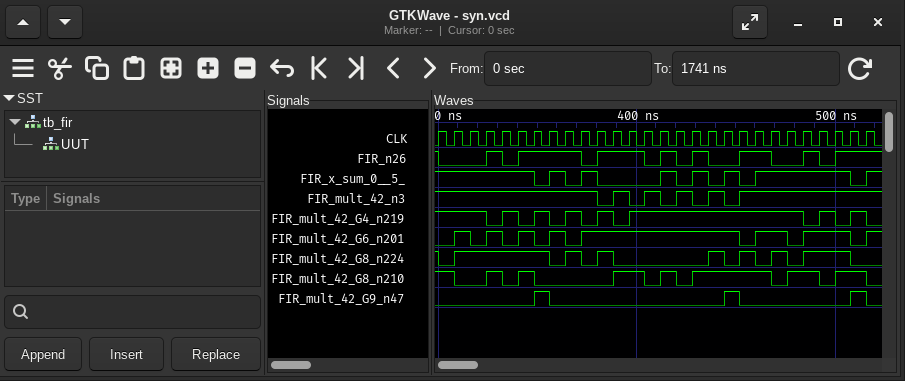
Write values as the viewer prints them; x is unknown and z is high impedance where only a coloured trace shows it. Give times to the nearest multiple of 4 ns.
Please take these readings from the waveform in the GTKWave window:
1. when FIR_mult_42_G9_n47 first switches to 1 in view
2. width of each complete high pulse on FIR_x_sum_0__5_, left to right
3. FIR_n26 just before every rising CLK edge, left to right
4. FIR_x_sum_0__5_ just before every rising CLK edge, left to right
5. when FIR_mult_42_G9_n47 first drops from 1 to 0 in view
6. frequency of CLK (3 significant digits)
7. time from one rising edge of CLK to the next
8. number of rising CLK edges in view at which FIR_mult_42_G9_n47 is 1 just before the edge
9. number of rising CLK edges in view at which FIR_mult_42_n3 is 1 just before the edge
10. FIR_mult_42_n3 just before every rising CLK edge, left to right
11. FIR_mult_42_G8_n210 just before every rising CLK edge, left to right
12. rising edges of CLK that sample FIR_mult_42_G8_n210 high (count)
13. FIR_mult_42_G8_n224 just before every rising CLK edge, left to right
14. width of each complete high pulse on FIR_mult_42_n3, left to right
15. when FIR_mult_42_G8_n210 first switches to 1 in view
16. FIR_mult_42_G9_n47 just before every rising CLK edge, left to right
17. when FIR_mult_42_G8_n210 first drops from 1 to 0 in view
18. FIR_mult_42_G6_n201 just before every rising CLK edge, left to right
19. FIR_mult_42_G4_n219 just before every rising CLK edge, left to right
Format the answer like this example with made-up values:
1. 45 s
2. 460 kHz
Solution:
1. 348 ns
2. 8 ns, 8 ns, 8 ns, 8 ns, 8 ns, 48 ns
3. 1 0 0 0 1 0 1 1 1 1 0 1 1 1 0 1 0 1 0 0 1 1 0 0 1 0 1 1
4. 1 1 1 1 1 1 1 0 1 0 1 0 0 0 0 1 0 1 0 1 0 1 1 1 1 1 1 0
5. 356 ns
6. 125 MHz
7. 8 ns
8. 3
9. 23
10. 1 1 1 1 1 1 1 1 1 1 1 0 1 0 1 0 1 0 1 0 1 1 1 1 1 1 1 1
11. 1 1 0 0 1 0 1 0 0 0 0 0 1 1 0 1 0 1 1 1 1 1 0 1 1 0 1 1
12. 16
13. 1 0 1 1 1 1 1 1 0 1 0 1 0 0 0 0 0 0 1 0 1 0 1 0 1 1 1 0
14. 8 ns, 8 ns, 8 ns, 8 ns
15. 324 ns
16. 0 0 0 0 0 0 0 1 0 0 0 0 0 0 0 0 0 0 0 1 0 0 0 0 0 0 0 1
17. 308 ns
18. 0 0 1 0 1 0 1 0 1 0 1 1 1 1 1 1 1 1 1 1 0 1 1 0 1 1 1 0
19. 1 1 1 1 0 1 0 1 0 1 0 1 0 1 1 1 1 1 1 1 1 1 1 1 0 1 0 1
